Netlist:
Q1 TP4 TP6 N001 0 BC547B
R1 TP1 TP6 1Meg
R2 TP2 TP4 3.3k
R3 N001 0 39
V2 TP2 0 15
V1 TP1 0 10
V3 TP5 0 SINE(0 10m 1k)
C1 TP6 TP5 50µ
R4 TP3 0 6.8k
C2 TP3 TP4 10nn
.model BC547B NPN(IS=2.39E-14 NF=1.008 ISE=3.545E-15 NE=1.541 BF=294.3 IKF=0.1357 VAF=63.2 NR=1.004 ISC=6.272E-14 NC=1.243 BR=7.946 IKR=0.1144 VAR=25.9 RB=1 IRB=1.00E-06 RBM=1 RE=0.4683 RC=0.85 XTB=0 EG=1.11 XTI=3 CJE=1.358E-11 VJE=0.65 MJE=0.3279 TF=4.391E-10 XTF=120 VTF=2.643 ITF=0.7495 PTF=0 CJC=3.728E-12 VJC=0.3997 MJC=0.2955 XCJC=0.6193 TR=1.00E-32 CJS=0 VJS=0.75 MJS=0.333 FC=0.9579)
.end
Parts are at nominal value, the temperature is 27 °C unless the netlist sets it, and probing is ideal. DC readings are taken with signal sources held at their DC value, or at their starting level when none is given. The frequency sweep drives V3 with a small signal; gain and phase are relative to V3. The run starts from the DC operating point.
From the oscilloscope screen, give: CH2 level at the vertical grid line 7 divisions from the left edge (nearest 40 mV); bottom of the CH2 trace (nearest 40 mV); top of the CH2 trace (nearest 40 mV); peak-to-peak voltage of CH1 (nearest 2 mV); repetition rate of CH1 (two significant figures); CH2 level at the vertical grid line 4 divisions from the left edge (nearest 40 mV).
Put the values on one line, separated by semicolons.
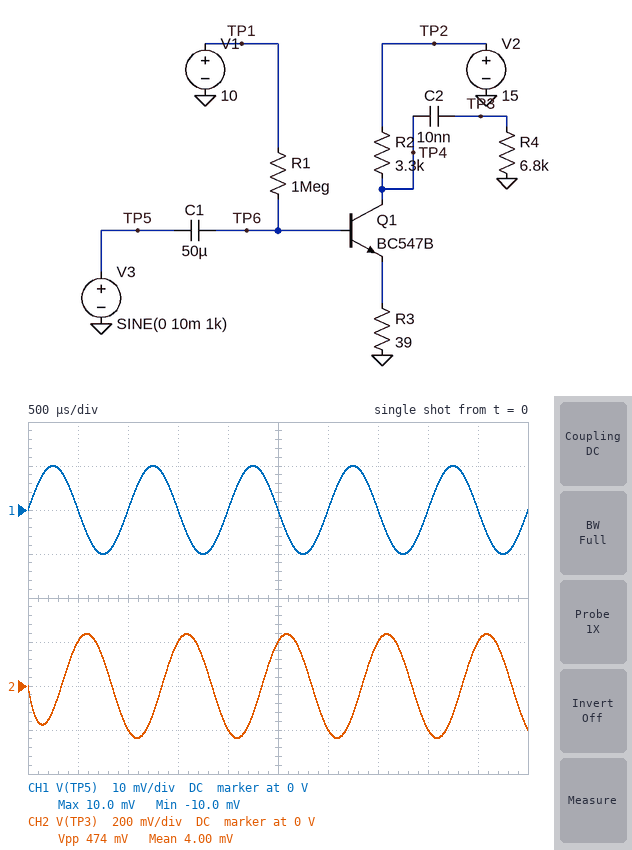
200 mV; -240 mV; 240 mV; 20 mV; 1.0 kHz; -200 mV
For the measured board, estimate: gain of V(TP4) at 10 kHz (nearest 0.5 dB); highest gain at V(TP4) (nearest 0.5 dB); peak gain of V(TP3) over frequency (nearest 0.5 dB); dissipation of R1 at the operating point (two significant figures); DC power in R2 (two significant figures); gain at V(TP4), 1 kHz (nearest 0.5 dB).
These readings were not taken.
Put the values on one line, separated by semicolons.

33.0 dB; 36.5 dB; 33.0 dB; 85 µW; 26 mW; 35.5 dB
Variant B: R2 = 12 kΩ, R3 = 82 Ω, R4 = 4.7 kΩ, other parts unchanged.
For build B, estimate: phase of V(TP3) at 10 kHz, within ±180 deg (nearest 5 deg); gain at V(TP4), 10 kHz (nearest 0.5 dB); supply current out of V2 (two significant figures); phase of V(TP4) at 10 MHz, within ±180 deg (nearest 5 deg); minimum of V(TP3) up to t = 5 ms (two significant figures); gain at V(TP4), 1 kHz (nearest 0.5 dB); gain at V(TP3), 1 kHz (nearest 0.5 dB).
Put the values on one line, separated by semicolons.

-165 deg; 23.0 dB; 1.2 mA; 90 deg; -210 mV; 25.5 dB; 14.5 dB
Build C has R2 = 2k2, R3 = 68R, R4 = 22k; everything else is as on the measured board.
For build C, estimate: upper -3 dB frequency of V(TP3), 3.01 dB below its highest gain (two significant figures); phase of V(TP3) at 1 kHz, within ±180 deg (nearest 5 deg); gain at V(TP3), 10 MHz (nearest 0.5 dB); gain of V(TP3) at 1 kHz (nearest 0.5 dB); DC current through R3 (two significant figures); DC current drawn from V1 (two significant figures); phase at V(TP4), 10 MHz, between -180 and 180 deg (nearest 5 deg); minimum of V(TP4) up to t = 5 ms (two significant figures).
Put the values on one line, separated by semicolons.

49 MHz; -145 deg; 28.0 dB; 26.5 dB; 2.9 mA; 9.1 µA; 165 deg; 8.4 V
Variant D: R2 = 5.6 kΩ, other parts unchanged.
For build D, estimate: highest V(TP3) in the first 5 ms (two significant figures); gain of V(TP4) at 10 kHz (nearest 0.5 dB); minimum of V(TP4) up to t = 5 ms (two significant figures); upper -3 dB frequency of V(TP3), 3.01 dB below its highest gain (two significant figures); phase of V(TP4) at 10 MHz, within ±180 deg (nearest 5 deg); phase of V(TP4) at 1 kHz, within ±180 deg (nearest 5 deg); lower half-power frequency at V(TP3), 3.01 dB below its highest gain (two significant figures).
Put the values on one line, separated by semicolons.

330 mV; 35.5 dB; 170 mV; 12 MHz; 135 deg; 165 deg; 1.3 kHz
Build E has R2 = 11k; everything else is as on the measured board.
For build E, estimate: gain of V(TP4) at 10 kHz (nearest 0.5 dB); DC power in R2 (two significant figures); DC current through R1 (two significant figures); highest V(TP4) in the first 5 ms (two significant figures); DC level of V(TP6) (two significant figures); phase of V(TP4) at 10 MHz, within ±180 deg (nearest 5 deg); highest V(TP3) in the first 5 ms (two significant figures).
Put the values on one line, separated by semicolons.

27.5 dB; 20 mW; 9.3 µA; 1.6 V; 700 mV; 95 deg; 370 mV
